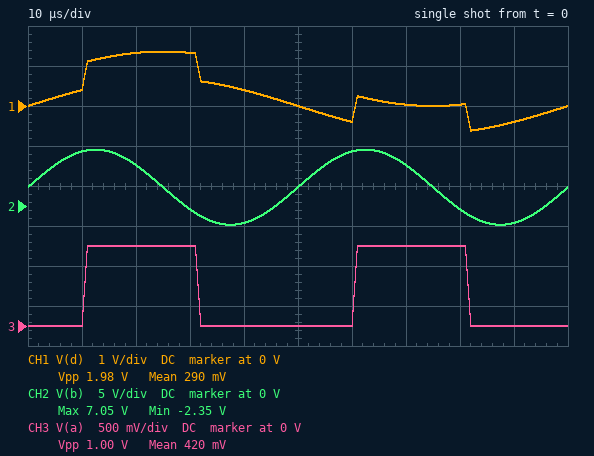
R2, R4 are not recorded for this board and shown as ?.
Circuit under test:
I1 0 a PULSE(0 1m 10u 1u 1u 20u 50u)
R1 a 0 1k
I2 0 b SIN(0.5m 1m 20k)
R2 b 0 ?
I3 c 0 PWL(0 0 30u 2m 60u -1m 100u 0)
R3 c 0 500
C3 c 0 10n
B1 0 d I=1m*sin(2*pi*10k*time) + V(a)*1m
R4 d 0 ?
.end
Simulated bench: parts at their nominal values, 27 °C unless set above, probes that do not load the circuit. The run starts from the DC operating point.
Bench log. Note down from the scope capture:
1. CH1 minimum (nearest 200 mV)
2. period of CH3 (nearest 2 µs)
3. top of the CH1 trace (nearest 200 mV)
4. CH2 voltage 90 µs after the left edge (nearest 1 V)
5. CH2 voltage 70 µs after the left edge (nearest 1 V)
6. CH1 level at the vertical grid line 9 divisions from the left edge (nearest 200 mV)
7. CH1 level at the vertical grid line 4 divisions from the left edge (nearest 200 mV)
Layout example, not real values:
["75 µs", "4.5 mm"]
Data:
["-600 mV", "50 µs", "1.4 V", "-2 V", "5 V", "-400 mV", "400 mV"]
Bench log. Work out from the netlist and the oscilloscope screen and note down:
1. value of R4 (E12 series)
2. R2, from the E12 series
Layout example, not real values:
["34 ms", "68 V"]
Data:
["680 Ω", "4.7 kΩ"]
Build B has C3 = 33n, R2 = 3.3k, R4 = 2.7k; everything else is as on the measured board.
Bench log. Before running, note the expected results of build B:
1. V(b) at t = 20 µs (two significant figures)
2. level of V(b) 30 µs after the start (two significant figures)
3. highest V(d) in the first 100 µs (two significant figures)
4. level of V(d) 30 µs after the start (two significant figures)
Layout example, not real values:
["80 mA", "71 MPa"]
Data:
["3.6 V", "-290 mV", "5.4 V", "5.3 V"]
